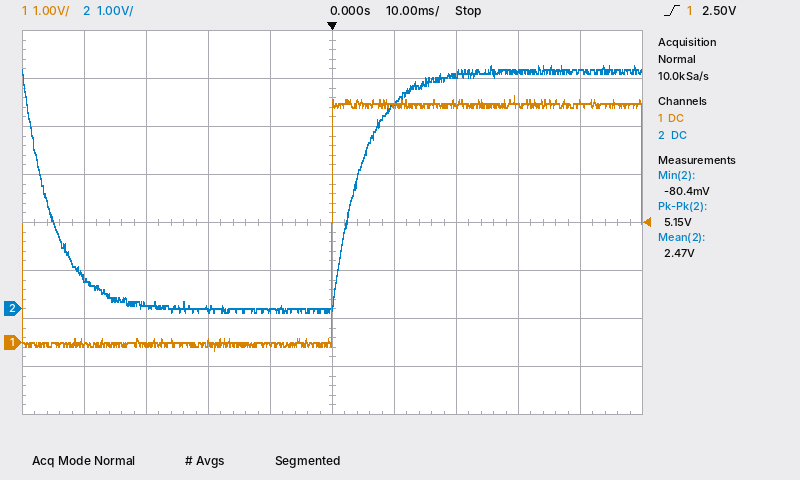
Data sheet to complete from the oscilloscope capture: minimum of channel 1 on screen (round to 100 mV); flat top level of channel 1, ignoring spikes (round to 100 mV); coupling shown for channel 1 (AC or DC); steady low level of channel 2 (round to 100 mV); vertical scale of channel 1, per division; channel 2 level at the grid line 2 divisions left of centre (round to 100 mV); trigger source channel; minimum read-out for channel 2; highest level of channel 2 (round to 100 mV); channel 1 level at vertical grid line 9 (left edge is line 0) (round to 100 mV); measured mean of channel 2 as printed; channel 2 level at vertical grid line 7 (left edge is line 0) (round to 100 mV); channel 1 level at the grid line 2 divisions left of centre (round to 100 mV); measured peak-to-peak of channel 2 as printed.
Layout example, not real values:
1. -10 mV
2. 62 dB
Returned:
1. -200 mV
2. 5.0 V
3. DC
4. 0.0 V
5. 1 V
6. 0.0 V
7. channel 1
8. -80.4 mV
9. 5.1 V
10. 5.0 V
11. 2.47 V
12. 4.9 V
13. 0.0 V
14. 5.15 V
